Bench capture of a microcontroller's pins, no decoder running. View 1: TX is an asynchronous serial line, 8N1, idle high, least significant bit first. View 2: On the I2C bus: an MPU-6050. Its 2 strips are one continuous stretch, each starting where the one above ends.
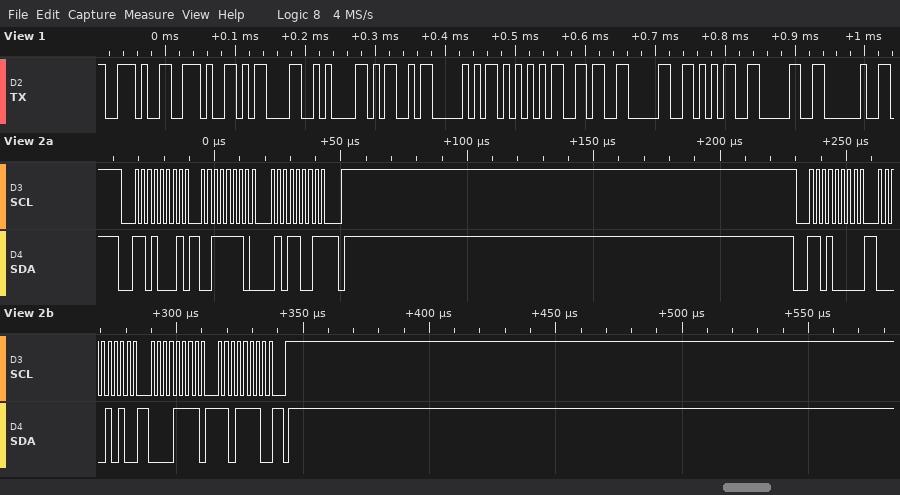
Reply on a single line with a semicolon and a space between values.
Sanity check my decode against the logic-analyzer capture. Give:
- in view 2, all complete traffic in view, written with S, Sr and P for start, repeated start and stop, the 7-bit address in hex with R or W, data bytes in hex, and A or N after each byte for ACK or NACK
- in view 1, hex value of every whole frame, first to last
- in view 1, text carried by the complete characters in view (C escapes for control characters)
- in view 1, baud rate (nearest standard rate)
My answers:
S 68R A 3E A 59 N P S 68W A 0A A 0F A DE A P; 2E 2E 0D 0A 4D 50 55 36 30 35 30 20; "..\r\nMPU6050 "; 115200 baud
